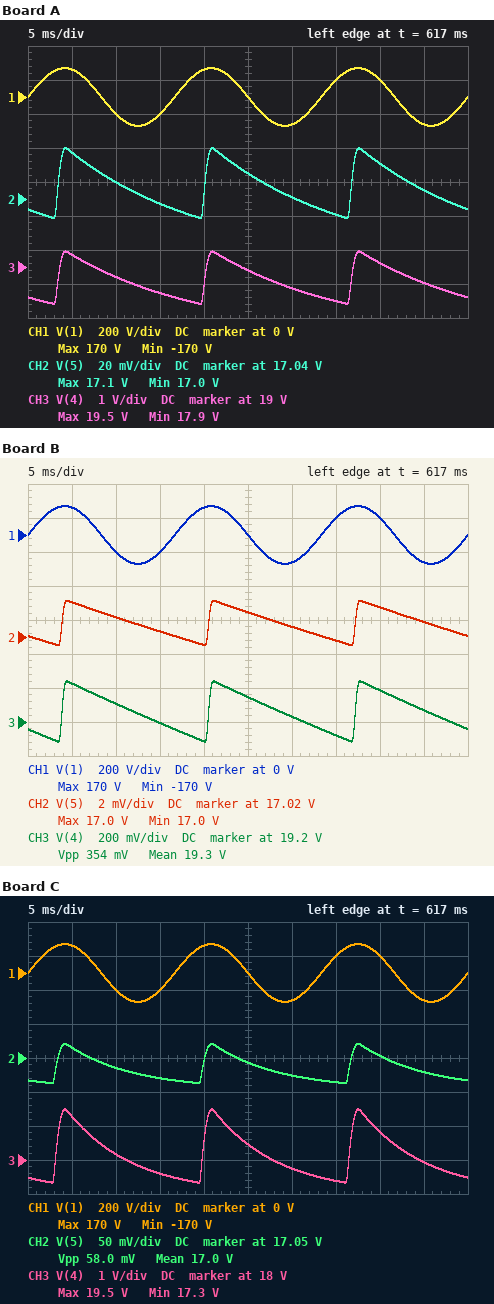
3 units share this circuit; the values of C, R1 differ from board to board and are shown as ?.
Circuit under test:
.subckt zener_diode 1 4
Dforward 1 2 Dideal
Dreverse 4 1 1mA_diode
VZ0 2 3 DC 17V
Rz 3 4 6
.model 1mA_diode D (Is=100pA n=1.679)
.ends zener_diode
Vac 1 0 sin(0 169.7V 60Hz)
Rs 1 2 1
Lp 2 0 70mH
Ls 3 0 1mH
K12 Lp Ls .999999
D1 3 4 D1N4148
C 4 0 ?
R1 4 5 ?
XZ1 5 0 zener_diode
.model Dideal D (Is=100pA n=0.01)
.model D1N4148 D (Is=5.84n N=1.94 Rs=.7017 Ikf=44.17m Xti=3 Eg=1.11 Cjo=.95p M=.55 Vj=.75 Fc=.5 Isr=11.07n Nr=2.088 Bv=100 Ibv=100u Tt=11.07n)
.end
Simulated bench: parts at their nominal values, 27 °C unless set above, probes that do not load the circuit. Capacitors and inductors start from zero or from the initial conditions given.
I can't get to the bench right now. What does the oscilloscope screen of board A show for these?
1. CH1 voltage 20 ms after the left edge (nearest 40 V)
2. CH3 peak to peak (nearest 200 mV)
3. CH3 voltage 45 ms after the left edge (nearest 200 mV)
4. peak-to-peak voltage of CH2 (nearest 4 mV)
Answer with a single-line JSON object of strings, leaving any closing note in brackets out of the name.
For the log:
{"CH1 voltage 20 ms after the left edge": "160 V", "CH3 peak to peak": "1.6 V", "CH3 voltage 45 ms after the left edge": "18.6 V", "peak-to-peak voltage of CH2": "40 mV"}
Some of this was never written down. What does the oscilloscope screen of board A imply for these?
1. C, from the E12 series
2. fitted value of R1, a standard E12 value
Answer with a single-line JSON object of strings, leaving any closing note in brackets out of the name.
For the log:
{"C, from the E12 series": "68 µF", "fitted value of R1, a standard E12 value": "220 Ω"}
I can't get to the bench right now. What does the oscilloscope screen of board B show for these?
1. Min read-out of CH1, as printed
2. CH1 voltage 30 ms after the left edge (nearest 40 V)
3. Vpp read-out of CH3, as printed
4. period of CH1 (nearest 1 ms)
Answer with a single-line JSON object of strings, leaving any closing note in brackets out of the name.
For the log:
{"Min read-out of CH1, as printed": "-170 V", "CH1 voltage 30 ms after the left edge": "-160 V", "Vpp read-out of CH3, as printed": "354 mV", "period of CH1": "17 ms"}
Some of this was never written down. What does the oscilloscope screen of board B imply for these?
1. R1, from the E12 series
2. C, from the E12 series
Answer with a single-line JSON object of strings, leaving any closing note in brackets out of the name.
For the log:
{"R1, from the E12 series": "820 Ω", "C, from the E12 series": "120 µF"}
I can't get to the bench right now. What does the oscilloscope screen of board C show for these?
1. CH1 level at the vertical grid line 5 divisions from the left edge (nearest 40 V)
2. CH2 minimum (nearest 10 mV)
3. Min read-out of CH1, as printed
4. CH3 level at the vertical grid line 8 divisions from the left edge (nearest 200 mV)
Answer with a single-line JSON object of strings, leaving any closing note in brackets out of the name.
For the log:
{"CH1 level at the vertical grid line 5 divisions from the left edge": "0 V", "CH2 minimum": "17.01 V", "Min read-out of CH1, as printed": "-170 V", "CH3 level at the vertical grid line 8 divisions from the left edge": "18.8 V"}
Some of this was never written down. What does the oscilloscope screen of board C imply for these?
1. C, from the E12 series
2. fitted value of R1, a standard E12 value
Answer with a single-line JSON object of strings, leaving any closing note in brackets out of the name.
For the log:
{"C, from the E12 series": "33 µF", "fitted value of R1, a standard E12 value": "220 Ω"}
